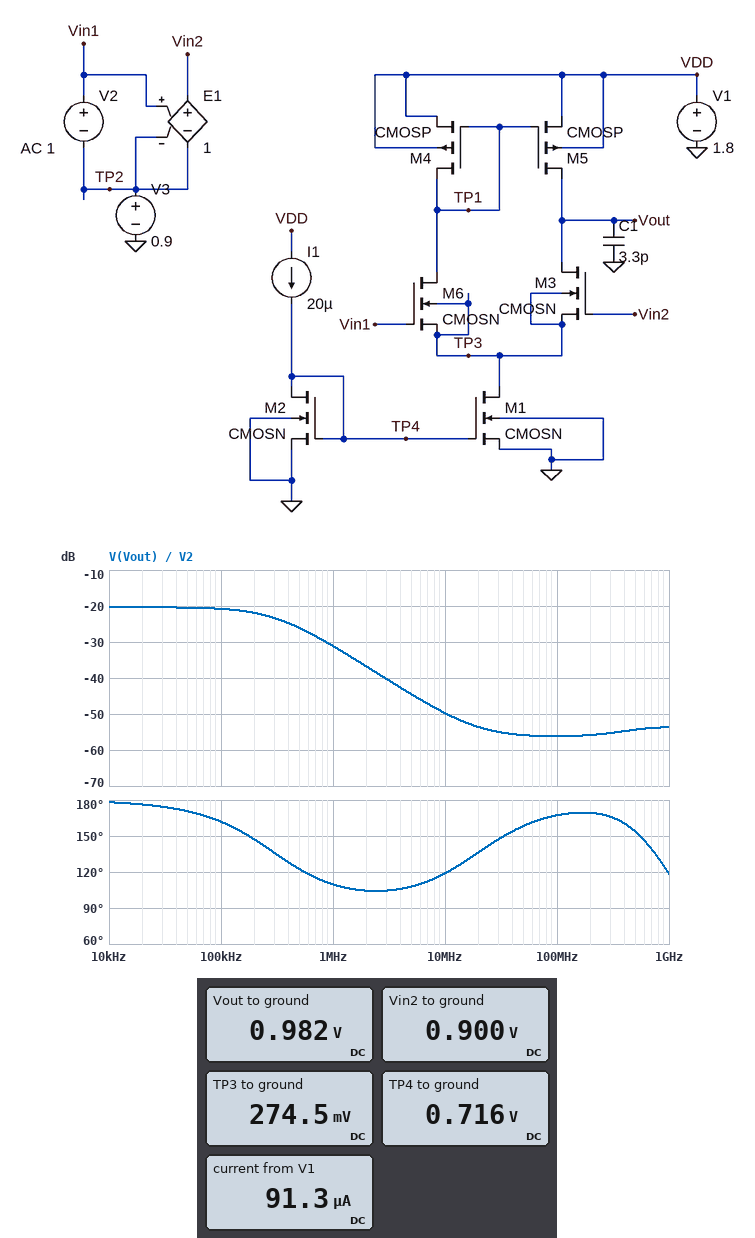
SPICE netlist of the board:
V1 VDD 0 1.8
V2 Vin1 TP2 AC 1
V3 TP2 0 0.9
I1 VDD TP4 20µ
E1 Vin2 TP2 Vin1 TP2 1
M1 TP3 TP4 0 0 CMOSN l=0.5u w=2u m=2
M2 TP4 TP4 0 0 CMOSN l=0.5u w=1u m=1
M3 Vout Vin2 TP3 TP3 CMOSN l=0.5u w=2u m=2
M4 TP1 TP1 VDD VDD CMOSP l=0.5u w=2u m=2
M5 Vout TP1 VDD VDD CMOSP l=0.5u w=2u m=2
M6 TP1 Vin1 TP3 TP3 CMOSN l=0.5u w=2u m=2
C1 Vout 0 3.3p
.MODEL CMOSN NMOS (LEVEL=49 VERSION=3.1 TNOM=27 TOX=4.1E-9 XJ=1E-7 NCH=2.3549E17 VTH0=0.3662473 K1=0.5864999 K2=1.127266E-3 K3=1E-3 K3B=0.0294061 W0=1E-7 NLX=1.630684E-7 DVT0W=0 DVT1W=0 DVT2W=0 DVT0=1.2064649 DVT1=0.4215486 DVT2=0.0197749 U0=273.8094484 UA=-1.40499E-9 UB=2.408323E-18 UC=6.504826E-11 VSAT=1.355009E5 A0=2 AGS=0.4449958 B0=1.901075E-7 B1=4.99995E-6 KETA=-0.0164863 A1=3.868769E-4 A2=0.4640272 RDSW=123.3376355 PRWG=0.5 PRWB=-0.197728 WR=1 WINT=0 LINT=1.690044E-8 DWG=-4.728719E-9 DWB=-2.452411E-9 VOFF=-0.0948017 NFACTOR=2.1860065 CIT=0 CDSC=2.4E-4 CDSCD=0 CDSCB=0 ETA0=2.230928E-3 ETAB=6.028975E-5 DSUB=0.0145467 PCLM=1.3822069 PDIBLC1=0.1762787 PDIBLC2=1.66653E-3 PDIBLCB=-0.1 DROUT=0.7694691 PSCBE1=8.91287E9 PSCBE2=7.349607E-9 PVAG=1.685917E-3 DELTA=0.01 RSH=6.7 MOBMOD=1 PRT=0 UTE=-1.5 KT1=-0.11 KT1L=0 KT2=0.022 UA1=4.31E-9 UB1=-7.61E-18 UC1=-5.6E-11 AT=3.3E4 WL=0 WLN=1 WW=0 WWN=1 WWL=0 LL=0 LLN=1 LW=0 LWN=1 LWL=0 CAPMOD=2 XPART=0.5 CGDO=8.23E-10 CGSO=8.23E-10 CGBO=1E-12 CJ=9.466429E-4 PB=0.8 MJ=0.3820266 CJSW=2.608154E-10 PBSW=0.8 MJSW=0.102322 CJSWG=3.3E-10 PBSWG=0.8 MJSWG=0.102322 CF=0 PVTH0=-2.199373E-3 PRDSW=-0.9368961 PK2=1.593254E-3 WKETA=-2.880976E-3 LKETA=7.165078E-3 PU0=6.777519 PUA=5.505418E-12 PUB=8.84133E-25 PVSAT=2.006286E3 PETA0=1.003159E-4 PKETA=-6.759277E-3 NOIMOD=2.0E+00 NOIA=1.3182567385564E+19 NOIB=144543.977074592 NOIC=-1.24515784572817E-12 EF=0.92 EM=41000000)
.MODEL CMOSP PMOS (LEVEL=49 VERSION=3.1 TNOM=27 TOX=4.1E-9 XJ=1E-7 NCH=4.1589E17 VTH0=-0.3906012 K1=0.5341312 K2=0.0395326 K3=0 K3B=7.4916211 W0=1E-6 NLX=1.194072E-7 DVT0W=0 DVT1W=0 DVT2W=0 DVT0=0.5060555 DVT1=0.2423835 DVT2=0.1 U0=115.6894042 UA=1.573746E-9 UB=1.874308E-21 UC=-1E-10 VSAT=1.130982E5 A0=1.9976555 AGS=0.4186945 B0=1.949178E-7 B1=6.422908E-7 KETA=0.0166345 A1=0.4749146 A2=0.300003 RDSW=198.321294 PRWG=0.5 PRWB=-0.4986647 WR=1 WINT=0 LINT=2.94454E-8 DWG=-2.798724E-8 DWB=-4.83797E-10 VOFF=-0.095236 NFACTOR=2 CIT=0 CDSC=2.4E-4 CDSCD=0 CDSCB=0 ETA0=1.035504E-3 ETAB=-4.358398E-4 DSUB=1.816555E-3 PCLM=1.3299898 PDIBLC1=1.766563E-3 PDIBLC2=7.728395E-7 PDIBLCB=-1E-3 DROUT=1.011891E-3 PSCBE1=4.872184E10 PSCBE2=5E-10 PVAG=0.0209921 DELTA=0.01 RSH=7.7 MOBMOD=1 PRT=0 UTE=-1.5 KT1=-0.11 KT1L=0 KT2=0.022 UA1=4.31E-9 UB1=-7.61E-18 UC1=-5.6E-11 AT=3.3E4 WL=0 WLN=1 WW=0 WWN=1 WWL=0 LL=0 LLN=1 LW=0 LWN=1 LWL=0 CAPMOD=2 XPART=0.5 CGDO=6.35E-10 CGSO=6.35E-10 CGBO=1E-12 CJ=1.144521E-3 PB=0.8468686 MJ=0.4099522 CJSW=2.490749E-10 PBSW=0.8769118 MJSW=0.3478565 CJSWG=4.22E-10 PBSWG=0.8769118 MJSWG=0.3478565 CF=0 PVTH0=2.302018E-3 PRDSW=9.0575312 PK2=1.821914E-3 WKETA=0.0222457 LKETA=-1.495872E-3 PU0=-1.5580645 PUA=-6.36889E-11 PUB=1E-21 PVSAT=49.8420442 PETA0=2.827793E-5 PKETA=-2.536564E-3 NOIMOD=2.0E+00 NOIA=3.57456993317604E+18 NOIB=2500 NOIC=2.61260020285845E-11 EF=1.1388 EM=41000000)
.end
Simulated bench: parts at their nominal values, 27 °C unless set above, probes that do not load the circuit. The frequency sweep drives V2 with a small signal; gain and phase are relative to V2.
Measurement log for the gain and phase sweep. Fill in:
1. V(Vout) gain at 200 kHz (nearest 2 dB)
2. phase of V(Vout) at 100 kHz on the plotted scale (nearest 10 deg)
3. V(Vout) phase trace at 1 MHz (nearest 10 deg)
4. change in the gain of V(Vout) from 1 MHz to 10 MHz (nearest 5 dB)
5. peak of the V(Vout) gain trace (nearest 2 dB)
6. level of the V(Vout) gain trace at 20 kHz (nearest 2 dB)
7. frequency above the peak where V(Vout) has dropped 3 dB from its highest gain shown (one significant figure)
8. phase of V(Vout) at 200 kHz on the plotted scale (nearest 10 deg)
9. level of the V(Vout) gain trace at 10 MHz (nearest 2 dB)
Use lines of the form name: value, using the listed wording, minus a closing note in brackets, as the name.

V(Vout) gain at 200 kHz: -22 dB
phase of V(Vout) at 100 kHz on the plotted scale: 160 deg
V(Vout) phase trace at 1 MHz: 110 deg
change in the gain of V(Vout) from 1 MHz to 10 MHz: -20 dB
peak of the V(Vout) gain trace: -20 dB
level of the V(Vout) gain trace at 20 kHz: -20 dB
frequency above the peak where V(Vout) has dropped 3 dB from its highest gain shown: 300 kHz
phase of V(Vout) at 200 kHz on the plotted scale: 150 deg
level of the V(Vout) gain trace at 10 MHz: -50 dB
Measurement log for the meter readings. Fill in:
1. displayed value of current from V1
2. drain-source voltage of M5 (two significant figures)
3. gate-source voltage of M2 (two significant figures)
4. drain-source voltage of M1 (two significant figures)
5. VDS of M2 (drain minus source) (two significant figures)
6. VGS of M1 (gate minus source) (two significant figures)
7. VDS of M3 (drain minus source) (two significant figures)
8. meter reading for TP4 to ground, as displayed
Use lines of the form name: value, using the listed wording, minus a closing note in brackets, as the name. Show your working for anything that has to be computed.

displayed value of current from V1: 91.3 µA
drain-source voltage of M5: 982 mV - 1.8 V = -820 mV
gate-source voltage of M2: 716 mV = 720 mV
drain-source voltage of M1: 274.5 mV = 270 mV
VDS of M2 (drain minus source): 716 mV = 720 mV
VGS of M1 (gate minus source): 716 mV = 720 mV
VDS of M3 (drain minus source): 982 mV - 274.5 mV = 710 mV
meter reading for TP4 to ground, as displayed: 0.716 V
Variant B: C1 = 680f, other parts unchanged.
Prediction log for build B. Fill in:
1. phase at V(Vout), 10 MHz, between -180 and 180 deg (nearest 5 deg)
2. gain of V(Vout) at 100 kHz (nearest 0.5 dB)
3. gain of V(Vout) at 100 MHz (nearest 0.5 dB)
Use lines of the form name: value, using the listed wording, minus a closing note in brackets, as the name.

phase at V(Vout), 10 MHz, between -180 and 180 deg: 125 deg
gain of V(Vout) at 100 kHz: -20.5 dB
gain of V(Vout) at 100 MHz: -42.5 dB
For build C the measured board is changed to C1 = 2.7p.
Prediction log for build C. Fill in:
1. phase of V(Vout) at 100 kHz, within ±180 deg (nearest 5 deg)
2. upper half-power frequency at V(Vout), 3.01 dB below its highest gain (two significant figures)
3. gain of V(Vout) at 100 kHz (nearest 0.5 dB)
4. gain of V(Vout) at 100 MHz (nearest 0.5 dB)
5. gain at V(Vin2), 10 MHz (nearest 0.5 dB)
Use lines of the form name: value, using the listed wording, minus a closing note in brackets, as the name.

phase of V(Vout) at 100 kHz, within ±180 deg: 165 deg
upper half-power frequency at V(Vout), 3.01 dB below its highest gain: 370 kHz
gain of V(Vout) at 100 kHz: -20.5 dB
gain of V(Vout) at 100 MHz: -54.5 dB
gain at V(Vin2), 10 MHz: 0 dB
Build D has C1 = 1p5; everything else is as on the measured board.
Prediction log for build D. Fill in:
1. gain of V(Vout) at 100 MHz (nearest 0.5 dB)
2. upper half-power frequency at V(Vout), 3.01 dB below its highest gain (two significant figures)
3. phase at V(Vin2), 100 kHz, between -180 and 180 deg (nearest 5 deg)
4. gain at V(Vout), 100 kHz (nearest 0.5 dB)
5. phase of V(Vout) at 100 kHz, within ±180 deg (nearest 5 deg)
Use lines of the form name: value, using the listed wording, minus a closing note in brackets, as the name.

gain of V(Vout) at 100 MHz: -49.5 dB
upper half-power frequency at V(Vout), 3.01 dB below its highest gain: 660 kHz
phase at V(Vin2), 100 kHz, between -180 and 180 deg: 0 deg
gain at V(Vout), 100 kHz: -20.5 dB
phase of V(Vout) at 100 kHz, within ±180 deg: 170 deg
